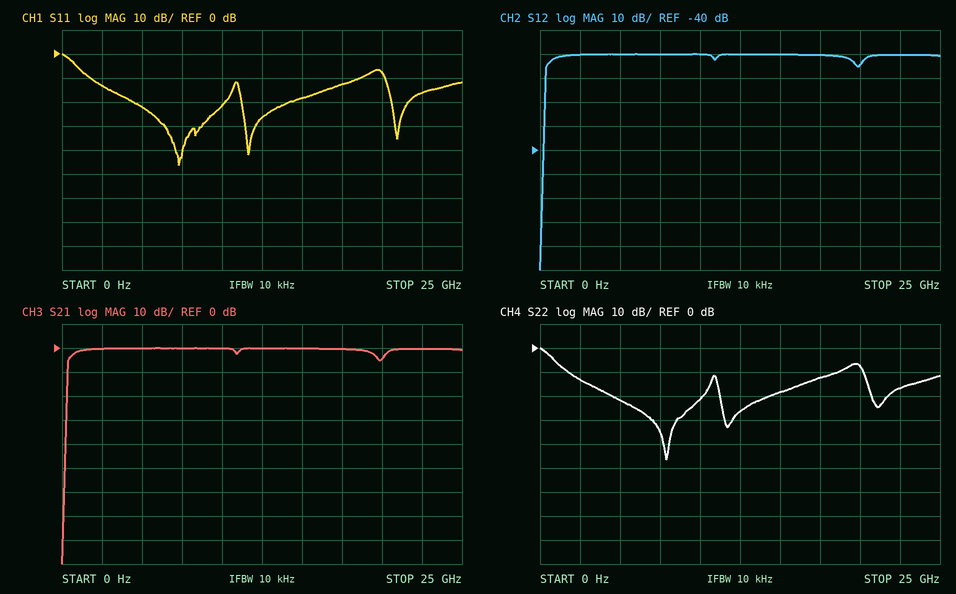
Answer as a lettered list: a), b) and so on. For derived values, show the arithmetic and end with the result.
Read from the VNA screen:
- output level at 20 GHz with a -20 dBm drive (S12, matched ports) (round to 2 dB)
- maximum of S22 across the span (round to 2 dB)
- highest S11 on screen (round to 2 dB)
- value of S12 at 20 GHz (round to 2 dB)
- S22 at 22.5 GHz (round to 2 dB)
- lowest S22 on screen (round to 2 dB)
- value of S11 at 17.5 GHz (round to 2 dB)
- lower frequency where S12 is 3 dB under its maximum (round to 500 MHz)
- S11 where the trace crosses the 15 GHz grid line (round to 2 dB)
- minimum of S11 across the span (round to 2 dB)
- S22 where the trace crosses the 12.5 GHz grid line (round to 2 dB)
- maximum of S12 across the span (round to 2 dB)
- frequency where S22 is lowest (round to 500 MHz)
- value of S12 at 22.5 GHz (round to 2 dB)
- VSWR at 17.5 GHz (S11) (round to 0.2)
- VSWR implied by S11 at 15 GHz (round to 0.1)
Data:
a) -20 dBm + (-4 dB) = -24 dBm
b) 0 dB
c) 0 dB
d) -4 dB
e) -16 dB
f) -46 dB
g) -12 dB
h) 500 MHz
i) -18 dB
j) -46 dB
k) -26 dB
l) 0 dB
m) 8.0 GHz
n) 0 dB
o) |Γ| = 10^(-12/20) = 0.2512; VSWR = (1 + 0.2512)/(1 − 0.2512) ≈ 1.67, so 1.6 to the nearest 0.2
p) |Γ| = 10^(-18/20) = 0.1259; VSWR = (1 + 0.1259)/(1 − 0.1259) ≈ 1.3
